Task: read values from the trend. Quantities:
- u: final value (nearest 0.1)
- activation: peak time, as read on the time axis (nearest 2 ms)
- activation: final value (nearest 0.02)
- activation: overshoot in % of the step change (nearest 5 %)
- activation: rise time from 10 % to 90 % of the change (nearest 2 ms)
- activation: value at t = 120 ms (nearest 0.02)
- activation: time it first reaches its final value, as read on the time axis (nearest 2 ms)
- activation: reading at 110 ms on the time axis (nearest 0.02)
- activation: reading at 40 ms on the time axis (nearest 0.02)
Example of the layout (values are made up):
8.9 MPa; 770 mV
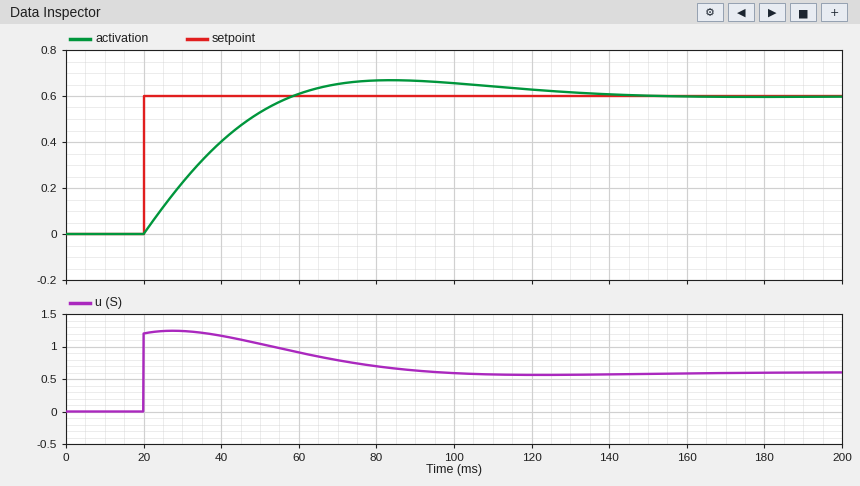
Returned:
0.6; 84 ms; 0.60; 10 %; 28 ms; 0.62; 58 ms; 0.64; 0.40
